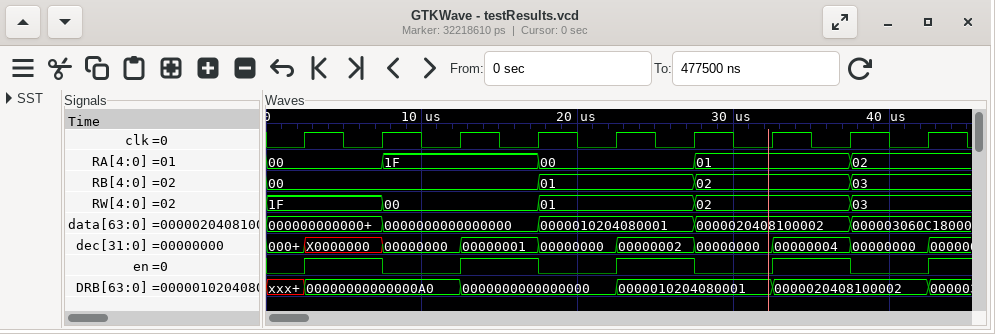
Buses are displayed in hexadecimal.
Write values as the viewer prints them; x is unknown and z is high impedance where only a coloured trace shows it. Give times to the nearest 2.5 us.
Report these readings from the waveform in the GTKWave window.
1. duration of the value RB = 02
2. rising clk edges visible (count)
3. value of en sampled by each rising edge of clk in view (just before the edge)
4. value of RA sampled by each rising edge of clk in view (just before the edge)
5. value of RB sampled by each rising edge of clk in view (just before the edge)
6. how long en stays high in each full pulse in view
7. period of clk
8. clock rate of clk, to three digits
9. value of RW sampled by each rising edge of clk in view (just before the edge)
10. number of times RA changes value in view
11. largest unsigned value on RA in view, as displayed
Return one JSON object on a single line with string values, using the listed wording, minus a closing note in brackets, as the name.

{"duration of the value RB = 02": "10 us", "rising clk edges visible": "9", "value of en sampled by each rising edge of clk in view": "0 1 0 1 0 1 0 1 0", "value of RA sampled by each rising edge of clk in view": "00, 00, 1F, 1F, 00, 00, 01, 01, 02", "value of RB sampled by each rising edge of clk in view": "00, 00, 00, 00, 01, 01, 02, 02, 03", "how long en stays high in each full pulse in view": "5 us, 5 us, 5 us, 5 us", "period of clk": "5 us", "clock rate of clk, to three digits": "200 kHz", "value of RW sampled by each rising edge of clk in view": "1F, 1F, 00, 00, 01, 01, 02, 02, 03", "number of times RA changes value in view": "4", "largest unsigned value on RA in view, as displayed": "1F"}
